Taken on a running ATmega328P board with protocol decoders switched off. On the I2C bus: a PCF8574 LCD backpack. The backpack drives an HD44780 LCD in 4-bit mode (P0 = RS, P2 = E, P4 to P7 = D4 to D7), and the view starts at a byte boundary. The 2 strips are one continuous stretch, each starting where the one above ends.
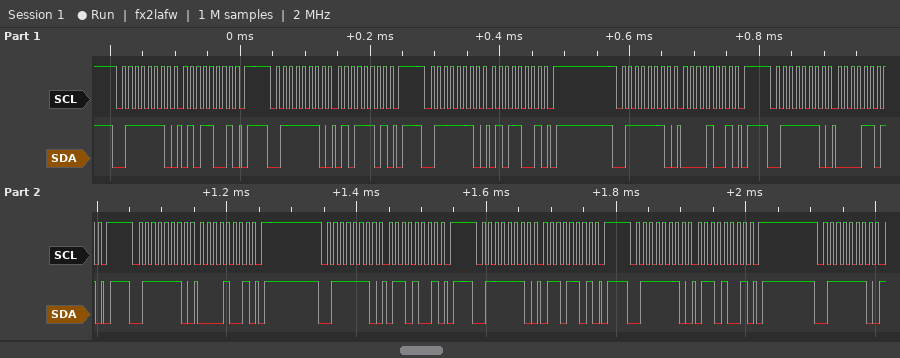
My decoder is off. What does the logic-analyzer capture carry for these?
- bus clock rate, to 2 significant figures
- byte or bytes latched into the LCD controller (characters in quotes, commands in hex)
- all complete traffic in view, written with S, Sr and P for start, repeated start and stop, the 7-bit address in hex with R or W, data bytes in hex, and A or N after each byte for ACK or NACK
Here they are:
100 kHz
'P'
S 3FW A 59 A P S 3FW A 5D A P S 3FW A 59 A P S 3FW A 09 A P S 3FW A 0D A P S 3FW A 09 A P S 3FW A 69 A P S 3FW A 6D A P S 3FW A 69 A P S 3FW A
